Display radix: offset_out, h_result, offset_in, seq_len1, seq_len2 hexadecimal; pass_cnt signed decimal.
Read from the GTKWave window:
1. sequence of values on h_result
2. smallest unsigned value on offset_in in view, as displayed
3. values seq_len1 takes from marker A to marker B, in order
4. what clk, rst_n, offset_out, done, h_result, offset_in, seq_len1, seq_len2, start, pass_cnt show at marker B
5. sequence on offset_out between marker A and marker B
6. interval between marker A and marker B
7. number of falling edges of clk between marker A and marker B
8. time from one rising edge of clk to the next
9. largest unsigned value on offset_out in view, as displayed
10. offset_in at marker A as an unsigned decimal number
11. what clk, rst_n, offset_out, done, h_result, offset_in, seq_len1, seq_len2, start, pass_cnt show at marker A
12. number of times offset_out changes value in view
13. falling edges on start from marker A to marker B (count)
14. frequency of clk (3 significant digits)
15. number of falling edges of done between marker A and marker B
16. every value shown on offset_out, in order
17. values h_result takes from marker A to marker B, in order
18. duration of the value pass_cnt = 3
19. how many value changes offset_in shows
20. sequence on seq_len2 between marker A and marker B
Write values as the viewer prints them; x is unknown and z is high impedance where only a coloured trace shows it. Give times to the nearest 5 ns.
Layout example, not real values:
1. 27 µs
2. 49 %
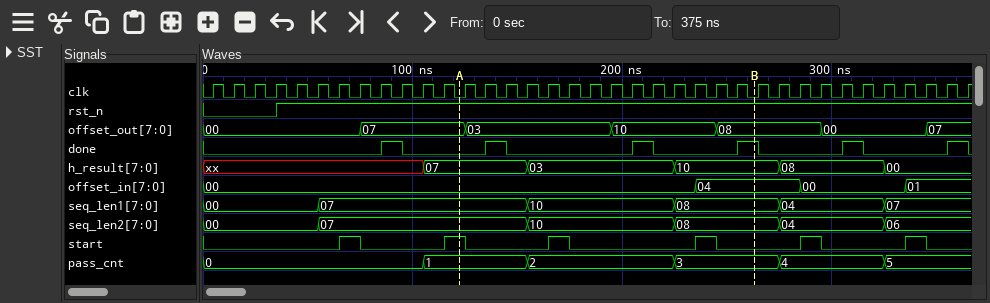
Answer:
1. xx, 07, 03, 10, 08, 00
2. 00
3. 07, 10, 08
4. clk=0, rst_n=1, offset_out=08, done=1, h_result=10, offset_in=04, seq_len1=08, seq_len2=08, start=0, pass_cnt=3
5. 07, 03, 10, 08
6. 140 ns
7. 14
8. 10 ns
9. 10
10. 0
11. clk=0, rst_n=1, offset_out=07, done=0, h_result=07, offset_in=00, seq_len1=07, seq_len2=07, start=1, pass_cnt=1
12. 6
13. 3
14. 100 MHz
15. 2
16. 00, 07, 03, 10, 08, 00, 07
17. 07, 03, 10
18. 50 ns
19. 3
20. 07, 10, 08
